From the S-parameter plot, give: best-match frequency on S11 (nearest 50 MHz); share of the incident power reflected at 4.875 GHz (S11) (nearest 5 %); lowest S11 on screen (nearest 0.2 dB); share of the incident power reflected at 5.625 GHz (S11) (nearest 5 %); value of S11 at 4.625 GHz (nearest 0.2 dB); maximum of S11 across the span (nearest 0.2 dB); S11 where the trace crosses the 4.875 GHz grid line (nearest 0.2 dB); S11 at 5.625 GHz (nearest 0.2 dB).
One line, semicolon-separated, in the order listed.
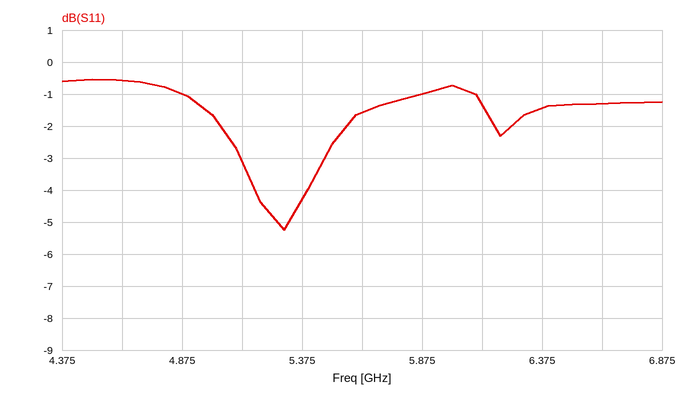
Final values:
5.30 GHz; 80 %; -5.2 dB; 70 %; -0.6 dB; -0.6 dB; -1.0 dB; -1.6 dB
